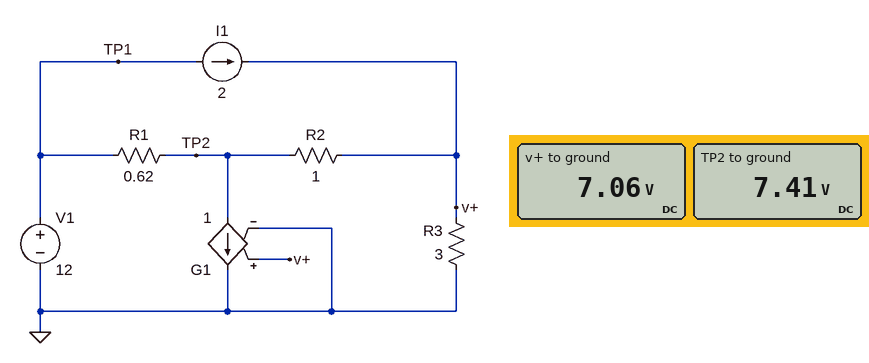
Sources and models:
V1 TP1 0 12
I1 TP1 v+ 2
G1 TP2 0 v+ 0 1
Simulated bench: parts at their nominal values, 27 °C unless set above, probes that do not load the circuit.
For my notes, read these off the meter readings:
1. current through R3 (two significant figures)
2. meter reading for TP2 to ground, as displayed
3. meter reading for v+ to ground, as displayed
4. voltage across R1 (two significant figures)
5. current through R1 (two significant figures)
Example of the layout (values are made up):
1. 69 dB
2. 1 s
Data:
1. 2.4 A
2. 7.41 V
3. 7.06 V
4. 4.6 V
5. 7.4 A
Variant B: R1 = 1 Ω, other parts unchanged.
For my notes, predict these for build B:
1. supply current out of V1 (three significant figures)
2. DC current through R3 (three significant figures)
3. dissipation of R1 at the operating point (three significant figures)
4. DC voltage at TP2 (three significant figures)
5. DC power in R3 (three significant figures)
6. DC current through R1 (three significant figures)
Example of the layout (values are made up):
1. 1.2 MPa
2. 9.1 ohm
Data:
1. 8.00 A
2. 2.00 A
3. 36.0 W
4. 6.00 V
5. 12.0 W
6. 6.00 A
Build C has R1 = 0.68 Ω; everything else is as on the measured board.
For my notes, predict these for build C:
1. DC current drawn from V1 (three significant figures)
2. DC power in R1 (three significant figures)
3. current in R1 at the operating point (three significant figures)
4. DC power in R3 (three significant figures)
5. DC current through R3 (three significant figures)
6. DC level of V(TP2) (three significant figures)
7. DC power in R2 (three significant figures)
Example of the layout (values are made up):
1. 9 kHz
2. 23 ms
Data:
1. 9.14 A
2. 34.7 W
3. 7.14 A
4. 15.7 W
5. 2.29 A
6. 7.14 V
7. 81.6 mW
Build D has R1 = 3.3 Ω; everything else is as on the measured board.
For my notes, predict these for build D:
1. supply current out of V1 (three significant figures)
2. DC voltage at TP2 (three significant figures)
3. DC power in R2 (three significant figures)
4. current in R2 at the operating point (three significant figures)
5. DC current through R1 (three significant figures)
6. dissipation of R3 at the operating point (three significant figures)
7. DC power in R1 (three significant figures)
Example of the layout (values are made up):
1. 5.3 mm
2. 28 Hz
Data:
1. 4.79 A
2. 2.79 V
3. 644 mW
4. 802 mA
5. 2.79 A
6. 4.30 W
7. 25.7 W
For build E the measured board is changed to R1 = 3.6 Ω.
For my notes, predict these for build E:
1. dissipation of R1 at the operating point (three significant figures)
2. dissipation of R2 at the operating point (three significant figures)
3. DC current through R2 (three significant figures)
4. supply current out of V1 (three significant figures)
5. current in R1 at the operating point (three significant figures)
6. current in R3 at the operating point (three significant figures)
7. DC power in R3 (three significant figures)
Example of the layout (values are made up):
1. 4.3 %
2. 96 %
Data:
1. 24.5 W
2. 719 mW
3. 848 mA
4. 4.61 A
5. 2.61 A
6. 1.15 A
7. 3.98 W
